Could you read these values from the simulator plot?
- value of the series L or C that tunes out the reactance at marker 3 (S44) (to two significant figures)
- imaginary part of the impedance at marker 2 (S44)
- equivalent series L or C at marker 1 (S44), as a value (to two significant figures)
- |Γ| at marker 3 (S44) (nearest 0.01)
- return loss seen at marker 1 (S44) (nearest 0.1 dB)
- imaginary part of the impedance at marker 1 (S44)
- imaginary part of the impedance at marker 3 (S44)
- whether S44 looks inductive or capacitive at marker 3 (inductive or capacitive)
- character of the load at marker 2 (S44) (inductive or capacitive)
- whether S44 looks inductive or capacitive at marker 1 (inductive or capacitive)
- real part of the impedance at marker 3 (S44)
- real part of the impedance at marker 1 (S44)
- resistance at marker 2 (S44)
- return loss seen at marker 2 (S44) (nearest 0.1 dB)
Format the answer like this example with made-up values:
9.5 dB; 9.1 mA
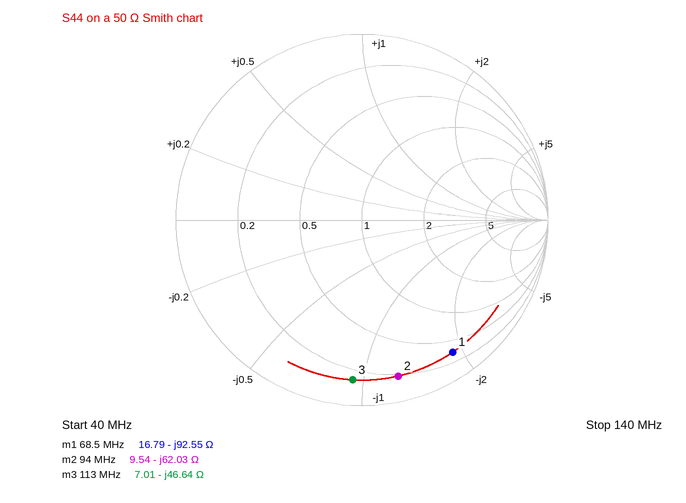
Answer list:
66 nH; -62.03 Ω; 25 pF; 0.86; 1.3 dB; -92.55 Ω; -46.64 Ω; capacitive; capacitive; capacitive; 7.01 Ω; 16.79 Ω; 9.54 Ω; 1.3 dB
